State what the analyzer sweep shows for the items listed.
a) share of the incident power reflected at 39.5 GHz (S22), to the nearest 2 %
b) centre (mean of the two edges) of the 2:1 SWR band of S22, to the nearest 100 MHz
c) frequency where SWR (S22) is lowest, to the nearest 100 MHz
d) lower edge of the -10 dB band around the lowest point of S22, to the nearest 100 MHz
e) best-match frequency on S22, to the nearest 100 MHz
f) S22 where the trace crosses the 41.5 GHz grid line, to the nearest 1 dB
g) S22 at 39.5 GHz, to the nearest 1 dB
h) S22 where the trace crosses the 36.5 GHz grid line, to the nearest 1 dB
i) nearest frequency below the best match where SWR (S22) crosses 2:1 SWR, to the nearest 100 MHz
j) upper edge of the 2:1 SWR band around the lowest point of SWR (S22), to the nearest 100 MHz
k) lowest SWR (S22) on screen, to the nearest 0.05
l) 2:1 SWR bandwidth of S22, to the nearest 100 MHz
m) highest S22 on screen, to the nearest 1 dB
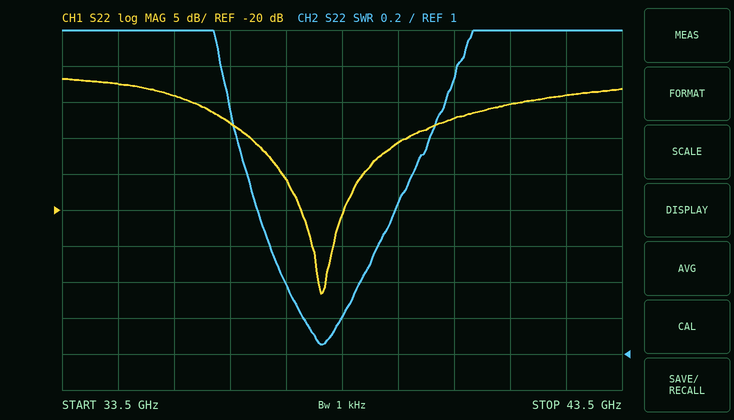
8 %
38.3 GHz
38.1 GHz
36.9 GHz
38.1 GHz
-5 dB
-11 dB
-8 dB
36.8 GHz
39.8 GHz
1.05
3.0 GHz
-2 dB
